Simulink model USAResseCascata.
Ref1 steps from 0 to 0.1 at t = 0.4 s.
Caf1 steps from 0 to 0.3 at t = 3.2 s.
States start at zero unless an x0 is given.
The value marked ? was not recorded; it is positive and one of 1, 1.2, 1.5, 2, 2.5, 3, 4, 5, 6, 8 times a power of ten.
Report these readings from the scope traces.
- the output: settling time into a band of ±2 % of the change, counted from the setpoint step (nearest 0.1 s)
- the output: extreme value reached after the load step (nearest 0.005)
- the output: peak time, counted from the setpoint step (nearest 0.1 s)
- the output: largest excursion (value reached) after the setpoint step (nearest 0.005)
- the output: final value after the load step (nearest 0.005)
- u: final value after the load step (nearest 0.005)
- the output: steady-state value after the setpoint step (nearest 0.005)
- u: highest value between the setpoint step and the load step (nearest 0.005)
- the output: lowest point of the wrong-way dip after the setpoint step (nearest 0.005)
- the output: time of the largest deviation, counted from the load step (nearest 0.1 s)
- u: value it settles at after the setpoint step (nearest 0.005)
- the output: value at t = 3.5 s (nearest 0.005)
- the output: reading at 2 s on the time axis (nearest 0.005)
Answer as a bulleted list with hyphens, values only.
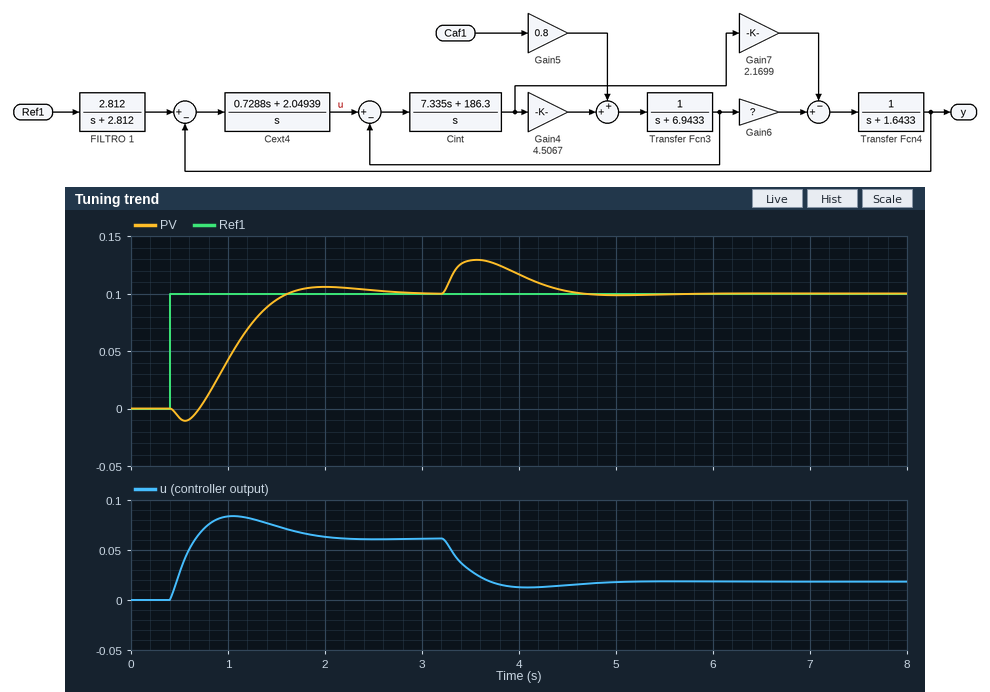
- 2.2 s
- 0.130
- 1.6 s
- 0.105
- 0.100
- 0.020
- 0.100
- 0.085
- -0.010
- 0.4 s
- 0.060
- 0.130
- 0.105
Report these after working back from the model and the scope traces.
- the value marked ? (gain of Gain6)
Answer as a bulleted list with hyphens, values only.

- 6
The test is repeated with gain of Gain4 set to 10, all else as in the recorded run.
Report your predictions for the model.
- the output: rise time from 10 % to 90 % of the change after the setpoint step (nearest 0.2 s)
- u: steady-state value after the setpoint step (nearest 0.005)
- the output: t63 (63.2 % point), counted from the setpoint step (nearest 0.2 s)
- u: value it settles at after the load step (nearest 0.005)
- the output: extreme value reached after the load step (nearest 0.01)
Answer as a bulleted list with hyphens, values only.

- 0.8 s
- 0.035
- 0.6 s
- 0.025
- 0.11
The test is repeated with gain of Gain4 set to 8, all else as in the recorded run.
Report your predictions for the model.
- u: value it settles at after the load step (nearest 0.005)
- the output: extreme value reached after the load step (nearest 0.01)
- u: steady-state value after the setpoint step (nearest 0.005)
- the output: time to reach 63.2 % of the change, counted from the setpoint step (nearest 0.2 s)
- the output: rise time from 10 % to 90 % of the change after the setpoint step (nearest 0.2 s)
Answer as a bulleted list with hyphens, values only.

- 0.025
- 0.11
- 0.040
- 0.6 s
- 0.8 s
